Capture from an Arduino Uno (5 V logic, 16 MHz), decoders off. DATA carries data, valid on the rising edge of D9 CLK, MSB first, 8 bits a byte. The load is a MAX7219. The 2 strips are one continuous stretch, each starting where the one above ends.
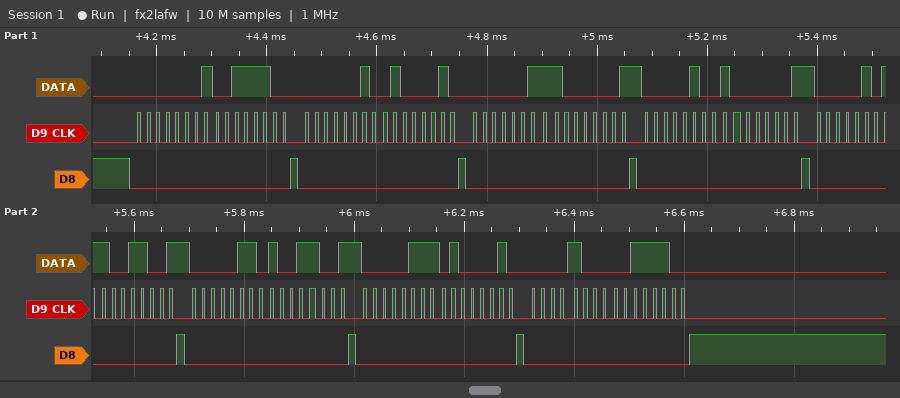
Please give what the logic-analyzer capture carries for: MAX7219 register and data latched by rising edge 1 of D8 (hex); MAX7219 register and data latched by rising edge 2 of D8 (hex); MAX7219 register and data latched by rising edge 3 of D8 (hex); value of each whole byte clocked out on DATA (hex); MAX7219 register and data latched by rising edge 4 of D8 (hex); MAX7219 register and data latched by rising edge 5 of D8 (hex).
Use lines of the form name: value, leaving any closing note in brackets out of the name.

MAX7219 register and data latched by rising edge 1 of D8: register 0x1, data 0x3C
MAX7219 register and data latched by rising edge 2 of D8: register 0x2, data 0x42
MAX7219 register and data latched by rising edge 3 of D8: register 0x3, data 0x81
value of each whole byte clocked out on DATA: 01 3C 02 42 03 81 04 81 05 99 06 99 07 42 08 3C
MAX7219 register and data latched by rising edge 4 of D8: register 0x4, data 0x81
MAX7219 register and data latched by rising edge 5 of D8: register 0x5, data 0x99
